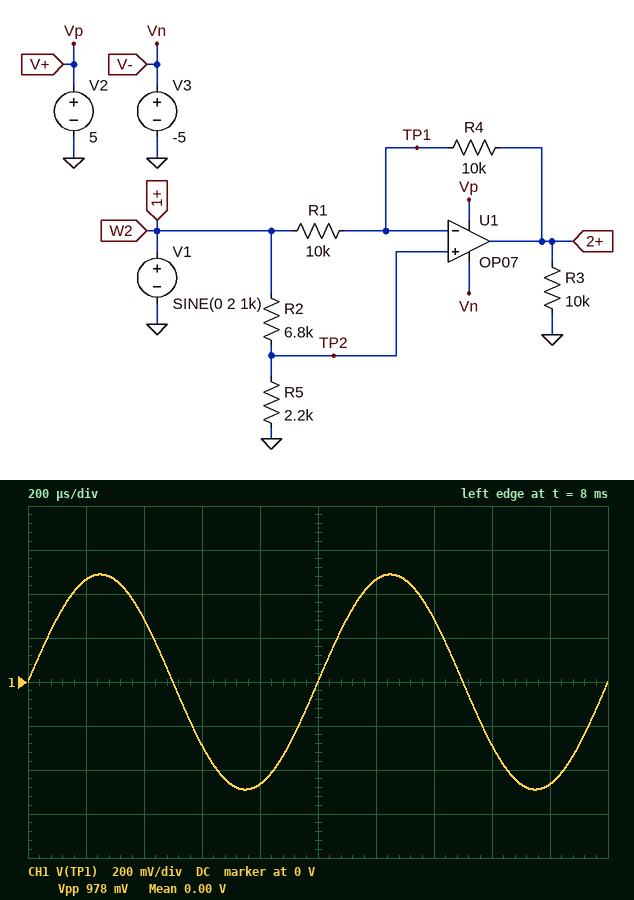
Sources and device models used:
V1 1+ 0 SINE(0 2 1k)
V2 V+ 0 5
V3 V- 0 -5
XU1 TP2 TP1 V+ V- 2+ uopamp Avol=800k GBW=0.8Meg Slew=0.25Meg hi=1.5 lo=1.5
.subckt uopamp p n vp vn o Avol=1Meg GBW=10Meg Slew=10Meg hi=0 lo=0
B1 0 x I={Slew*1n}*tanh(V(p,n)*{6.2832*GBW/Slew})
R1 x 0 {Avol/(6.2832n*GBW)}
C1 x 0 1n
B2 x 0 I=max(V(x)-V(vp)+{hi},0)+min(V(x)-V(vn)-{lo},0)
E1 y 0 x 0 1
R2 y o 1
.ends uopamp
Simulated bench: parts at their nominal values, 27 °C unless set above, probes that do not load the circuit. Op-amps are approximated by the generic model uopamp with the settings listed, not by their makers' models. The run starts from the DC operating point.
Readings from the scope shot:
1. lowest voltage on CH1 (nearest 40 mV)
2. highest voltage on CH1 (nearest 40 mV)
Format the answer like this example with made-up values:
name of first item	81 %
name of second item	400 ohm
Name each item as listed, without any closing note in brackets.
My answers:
lowest voltage on CH1	-480 mV
highest voltage on CH1	480 mV
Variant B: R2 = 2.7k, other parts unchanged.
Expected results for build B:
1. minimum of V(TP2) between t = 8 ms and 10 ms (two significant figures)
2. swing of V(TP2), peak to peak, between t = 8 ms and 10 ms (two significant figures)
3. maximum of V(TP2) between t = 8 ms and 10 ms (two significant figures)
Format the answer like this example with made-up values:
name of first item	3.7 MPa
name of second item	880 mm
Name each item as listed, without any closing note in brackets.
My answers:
minimum of V(TP2) between t = 8 ms and 10 ms	-900 mV
swing of V(TP2), peak to peak, between t = 8 ms and 10 ms	1.8 V
maximum of V(TP2) between t = 8 ms and 10 ms	900 mV
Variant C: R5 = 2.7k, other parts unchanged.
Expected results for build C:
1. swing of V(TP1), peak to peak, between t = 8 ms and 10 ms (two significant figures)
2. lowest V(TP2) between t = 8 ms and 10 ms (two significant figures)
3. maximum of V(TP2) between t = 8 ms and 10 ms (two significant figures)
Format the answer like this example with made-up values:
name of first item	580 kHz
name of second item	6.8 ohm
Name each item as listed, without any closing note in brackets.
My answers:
swing of V(TP1), peak to peak, between t = 8 ms and 10 ms	1.1 V
lowest V(TP2) between t = 8 ms and 10 ms	-570 mV
maximum of V(TP2) between t = 8 ms and 10 ms	570 mV
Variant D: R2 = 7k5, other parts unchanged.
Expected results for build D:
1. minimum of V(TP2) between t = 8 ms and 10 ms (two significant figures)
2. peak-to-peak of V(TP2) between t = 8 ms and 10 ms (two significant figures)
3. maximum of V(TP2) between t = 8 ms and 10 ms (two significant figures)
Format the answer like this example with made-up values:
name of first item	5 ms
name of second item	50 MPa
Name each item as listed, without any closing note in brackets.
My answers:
minimum of V(TP2) between t = 8 ms and 10 ms	-450 mV
peak-to-peak of V(TP2) between t = 8 ms and 10 ms	910 mV
maximum of V(TP2) between t = 8 ms and 10 ms	450 mV
